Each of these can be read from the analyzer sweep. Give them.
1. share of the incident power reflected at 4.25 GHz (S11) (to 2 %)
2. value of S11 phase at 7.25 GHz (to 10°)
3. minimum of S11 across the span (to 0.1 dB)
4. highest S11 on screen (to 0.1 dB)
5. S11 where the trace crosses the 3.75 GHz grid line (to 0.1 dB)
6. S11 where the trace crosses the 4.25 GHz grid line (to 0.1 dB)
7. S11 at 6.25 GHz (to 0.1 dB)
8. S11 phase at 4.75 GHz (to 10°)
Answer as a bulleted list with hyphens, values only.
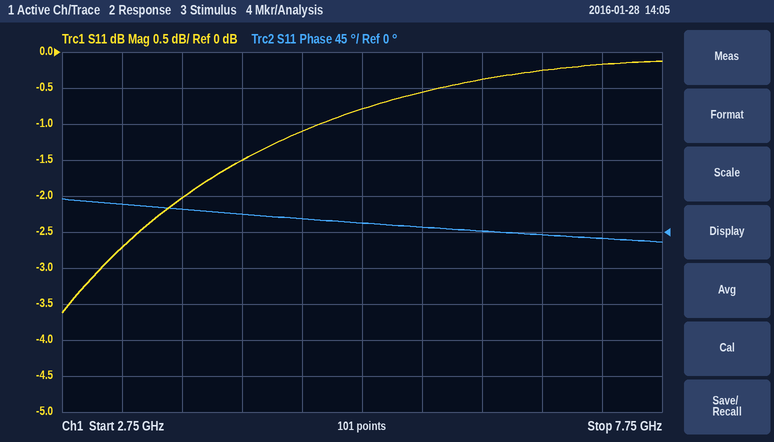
- 70 %
- -10°
- -3.6 dB
- -0.1 dB
- -2.0 dB
- -1.5 dB
- -0.4 dB
- 20°
